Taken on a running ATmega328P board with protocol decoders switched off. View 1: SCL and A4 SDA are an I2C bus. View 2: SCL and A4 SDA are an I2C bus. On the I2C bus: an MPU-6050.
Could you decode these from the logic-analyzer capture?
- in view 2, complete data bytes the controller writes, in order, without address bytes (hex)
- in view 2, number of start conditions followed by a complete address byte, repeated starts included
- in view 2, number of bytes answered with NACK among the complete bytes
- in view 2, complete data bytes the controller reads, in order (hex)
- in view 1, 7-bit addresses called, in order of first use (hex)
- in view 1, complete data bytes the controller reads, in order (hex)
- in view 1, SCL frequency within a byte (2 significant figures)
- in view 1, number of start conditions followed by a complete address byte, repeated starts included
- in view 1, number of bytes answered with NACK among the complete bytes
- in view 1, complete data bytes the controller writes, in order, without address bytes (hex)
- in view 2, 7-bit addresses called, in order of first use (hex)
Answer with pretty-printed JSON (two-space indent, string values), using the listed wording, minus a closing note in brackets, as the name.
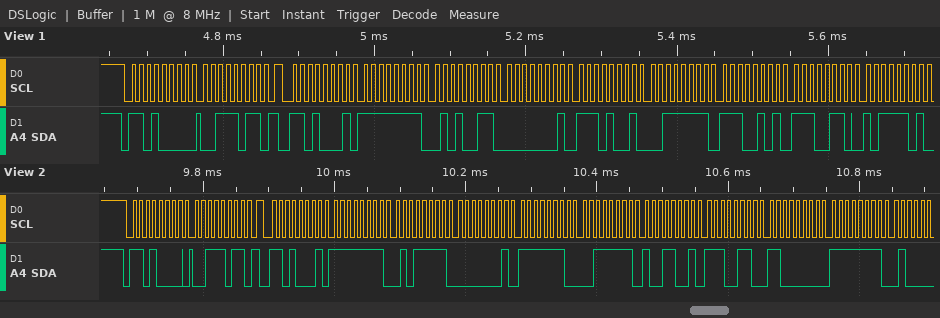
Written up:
{
  "in view 2, complete data bytes the controller writes, in order, without address bytes": "3B",
  "in view 2, number of start conditions followed by a complete address byte, repeated starts included": "2",
  "in view 2, number of bytes answered with NACK among the complete bytes": "0",
  "in view 2, complete data bytes the controller reads, in order": "FF 5F 01 FE 3F 99 E6 C0 FF",
  "in view 1, 7-bit addresses called, in order of first use": "0x68",
  "in view 1, complete data bytes the controller reads, in order": "FF 53 01 E9 3F E5 E6 BD",
  "in view 1, SCL frequency within a byte": "100 kHz",
  "in view 1, number of start conditions followed by a complete address byte, repeated starts included": "2",
  "in view 1, number of bytes answered with NACK among the complete bytes": "0",
  "in view 1, complete data bytes the controller writes, in order, without address bytes": "3B",
  "in view 2, 7-bit addresses called, in order of first use": "0x68"
}
